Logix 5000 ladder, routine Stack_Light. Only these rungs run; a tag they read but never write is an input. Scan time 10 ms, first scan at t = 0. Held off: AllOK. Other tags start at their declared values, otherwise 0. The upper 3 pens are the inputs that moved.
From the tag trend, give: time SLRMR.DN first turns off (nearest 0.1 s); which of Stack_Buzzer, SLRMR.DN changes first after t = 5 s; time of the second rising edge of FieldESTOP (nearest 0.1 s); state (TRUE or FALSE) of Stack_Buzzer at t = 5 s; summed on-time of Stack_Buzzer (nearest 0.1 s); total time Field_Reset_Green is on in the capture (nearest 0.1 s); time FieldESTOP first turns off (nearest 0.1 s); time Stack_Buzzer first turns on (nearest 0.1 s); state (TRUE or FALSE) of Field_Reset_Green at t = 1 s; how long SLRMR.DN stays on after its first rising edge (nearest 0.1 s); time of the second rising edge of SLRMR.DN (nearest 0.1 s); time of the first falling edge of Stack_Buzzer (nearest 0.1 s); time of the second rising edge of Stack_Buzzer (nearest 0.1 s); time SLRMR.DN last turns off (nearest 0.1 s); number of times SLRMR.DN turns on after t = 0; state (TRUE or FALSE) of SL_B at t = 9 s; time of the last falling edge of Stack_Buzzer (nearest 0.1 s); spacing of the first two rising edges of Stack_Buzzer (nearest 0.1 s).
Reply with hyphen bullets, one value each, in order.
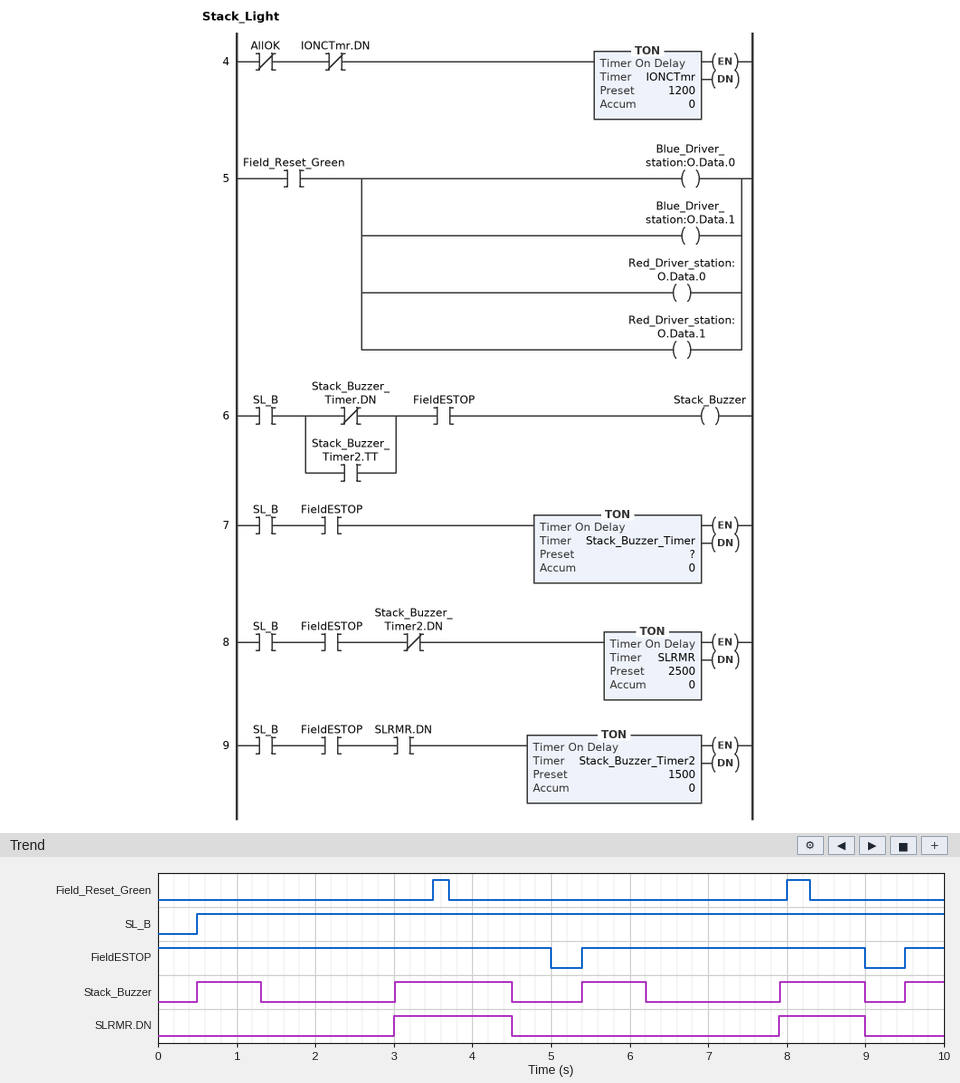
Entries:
- 4.5 s
- Stack_Buzzer
- 9.5 s
- FALSE
- 4.7 s
- 0.5 s
- 5.0 s
- 0.5 s
- FALSE
- 1.5 s
- 7.9 s
- 1.3 s
- 3.0 s
- 9.0 s
- 2
- TRUE
- 9.0 s
- 2.5 s
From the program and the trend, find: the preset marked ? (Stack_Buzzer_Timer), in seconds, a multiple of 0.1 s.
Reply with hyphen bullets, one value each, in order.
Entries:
- 0.8 s
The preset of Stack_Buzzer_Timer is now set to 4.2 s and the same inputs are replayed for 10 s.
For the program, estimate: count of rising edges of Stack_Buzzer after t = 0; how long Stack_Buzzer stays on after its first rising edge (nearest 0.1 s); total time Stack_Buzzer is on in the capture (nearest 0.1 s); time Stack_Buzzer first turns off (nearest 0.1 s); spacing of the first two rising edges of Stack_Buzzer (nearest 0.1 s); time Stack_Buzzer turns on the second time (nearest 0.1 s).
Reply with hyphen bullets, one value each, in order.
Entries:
- 3
- 4.2 s
- 8.3 s
- 4.7 s
- 4.9 s
- 5.4 s
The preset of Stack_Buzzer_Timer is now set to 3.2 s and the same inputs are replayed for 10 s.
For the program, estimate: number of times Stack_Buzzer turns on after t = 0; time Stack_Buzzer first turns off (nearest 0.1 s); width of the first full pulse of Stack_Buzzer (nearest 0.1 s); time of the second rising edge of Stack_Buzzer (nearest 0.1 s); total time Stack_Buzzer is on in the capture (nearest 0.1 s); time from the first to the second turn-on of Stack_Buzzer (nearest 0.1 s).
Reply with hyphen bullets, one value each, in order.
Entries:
- 3
- 4.5 s
- 4.0 s
- 5.4 s
- 8.1 s
- 4.9 s
